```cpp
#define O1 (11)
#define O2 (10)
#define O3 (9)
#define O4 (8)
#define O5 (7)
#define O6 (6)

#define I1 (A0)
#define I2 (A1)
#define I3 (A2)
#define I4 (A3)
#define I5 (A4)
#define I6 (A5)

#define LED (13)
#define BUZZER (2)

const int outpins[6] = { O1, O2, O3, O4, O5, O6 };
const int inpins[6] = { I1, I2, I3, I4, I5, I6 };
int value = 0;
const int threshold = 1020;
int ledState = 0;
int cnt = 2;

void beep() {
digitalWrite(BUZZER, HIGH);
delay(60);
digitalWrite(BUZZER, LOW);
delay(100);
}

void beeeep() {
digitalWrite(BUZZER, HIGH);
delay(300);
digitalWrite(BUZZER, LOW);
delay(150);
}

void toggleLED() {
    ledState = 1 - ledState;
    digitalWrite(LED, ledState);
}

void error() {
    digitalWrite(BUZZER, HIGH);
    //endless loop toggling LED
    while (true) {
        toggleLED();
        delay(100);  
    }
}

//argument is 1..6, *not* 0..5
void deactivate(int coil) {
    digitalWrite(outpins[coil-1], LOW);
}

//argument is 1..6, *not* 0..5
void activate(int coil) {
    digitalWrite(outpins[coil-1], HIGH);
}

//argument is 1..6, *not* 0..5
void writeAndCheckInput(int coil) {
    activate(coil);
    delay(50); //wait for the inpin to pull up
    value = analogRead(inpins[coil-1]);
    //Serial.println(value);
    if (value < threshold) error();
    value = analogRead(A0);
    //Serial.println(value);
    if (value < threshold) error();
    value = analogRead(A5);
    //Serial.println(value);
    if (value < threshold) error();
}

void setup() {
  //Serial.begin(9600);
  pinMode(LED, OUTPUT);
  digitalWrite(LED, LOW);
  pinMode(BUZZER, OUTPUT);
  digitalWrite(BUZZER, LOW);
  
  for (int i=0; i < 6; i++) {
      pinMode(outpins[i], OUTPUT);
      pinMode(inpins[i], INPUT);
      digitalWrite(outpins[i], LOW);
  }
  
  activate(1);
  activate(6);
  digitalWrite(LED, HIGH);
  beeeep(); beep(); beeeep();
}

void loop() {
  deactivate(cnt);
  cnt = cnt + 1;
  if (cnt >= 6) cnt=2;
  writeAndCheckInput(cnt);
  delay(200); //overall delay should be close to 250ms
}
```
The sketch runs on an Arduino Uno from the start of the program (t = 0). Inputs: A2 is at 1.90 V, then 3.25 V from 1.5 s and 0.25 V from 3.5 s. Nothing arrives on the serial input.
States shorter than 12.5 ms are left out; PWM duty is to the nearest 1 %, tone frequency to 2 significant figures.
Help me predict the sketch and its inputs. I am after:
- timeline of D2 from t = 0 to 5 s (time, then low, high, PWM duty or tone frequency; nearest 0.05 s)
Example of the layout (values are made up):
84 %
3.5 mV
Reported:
0 s high; 0.3 s low; 0.45 s high; 0.5 s low; 0.6 s high; 0.9 s low; 1.1 s high
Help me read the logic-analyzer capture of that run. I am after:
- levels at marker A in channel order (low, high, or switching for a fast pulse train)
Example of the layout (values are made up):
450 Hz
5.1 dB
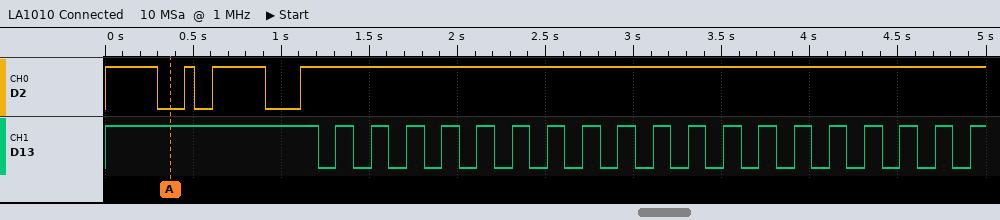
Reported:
D2 low, D13 high
